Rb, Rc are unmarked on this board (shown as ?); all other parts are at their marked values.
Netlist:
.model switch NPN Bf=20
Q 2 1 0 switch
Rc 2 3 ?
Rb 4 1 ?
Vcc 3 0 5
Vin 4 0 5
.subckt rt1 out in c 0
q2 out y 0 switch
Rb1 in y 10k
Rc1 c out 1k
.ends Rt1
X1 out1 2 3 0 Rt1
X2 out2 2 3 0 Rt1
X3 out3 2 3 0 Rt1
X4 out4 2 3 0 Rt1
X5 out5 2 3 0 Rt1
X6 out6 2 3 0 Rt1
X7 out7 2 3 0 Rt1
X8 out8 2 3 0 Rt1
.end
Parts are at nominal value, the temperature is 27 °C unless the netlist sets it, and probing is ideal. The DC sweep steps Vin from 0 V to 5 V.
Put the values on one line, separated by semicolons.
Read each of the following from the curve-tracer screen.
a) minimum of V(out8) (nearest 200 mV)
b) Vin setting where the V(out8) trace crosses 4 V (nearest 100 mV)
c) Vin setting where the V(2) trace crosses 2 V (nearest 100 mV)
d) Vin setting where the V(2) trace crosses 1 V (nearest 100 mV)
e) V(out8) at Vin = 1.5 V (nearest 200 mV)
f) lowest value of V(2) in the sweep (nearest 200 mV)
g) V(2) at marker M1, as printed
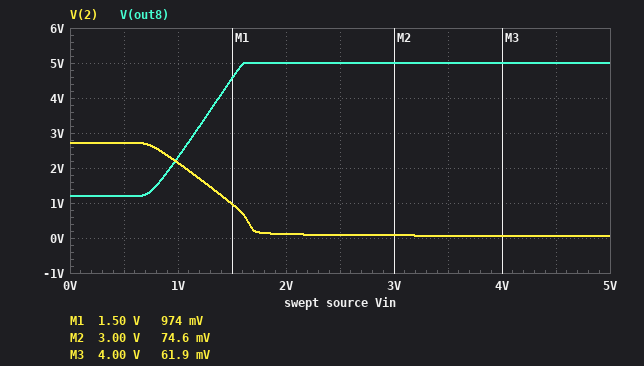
1.2 V; 1.4 V; 1.1 V; 1.5 V; 4.6 V; 0 V; 974 mV
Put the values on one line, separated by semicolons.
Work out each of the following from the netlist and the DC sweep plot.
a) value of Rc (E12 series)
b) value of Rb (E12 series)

1.5 kΩ; 5.6 kΩ
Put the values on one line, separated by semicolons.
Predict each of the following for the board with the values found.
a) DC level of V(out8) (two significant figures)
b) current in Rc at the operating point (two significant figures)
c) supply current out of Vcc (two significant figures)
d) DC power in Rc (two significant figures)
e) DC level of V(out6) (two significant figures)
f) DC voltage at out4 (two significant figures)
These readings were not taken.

5.0 V; 3.3 mA; 3.3 mA; 16 mW; 5.0 V; 5.0 V
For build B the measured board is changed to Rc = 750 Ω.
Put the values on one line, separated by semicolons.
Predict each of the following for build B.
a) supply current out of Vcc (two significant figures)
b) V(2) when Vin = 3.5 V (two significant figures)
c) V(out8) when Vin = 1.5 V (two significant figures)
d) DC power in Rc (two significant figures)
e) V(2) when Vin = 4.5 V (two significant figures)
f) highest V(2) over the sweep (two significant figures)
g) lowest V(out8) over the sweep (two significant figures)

6.6 mA; 100 mV; 2.1 V; 32 mW; 82 mV; 3.4 V; 150 mV
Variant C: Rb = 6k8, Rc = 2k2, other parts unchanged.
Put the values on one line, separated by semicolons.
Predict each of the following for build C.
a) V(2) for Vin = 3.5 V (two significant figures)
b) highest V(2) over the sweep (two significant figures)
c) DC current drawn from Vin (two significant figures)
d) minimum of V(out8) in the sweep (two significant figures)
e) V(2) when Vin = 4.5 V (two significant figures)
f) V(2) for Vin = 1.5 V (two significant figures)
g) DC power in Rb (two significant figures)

61 mV; 2.3 V; 620 µA; 2.0 V; 53 mV; 430 mV; 2.6 mW
